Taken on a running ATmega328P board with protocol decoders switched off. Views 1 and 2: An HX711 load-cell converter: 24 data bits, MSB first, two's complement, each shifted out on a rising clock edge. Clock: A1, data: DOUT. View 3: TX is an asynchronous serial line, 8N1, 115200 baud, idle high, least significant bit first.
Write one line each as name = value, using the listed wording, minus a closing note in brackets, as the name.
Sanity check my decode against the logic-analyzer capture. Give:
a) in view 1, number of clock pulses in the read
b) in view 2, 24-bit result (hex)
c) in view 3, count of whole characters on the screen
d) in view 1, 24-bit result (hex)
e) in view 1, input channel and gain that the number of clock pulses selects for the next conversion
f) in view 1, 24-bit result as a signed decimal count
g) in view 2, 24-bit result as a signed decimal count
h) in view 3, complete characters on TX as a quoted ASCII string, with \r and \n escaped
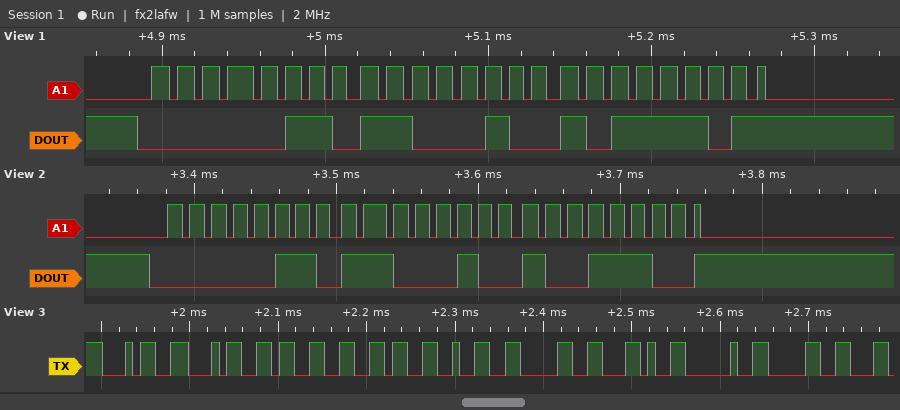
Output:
in view 1, number of clock pulses in the read = 25
in view 2, 24-bit result = 0x06C49C
in view 3, count of whole characters on the screen = 9
in view 1, 24-bit result = 0x06C4BD
in view 1, input channel and gain that the number of clock pulses selects for the next conversion = channel A, gain 128
in view 1, 24-bit result as a signed decimal count = 443581
in view 2, 24-bit result as a signed decimal count = 443548
in view 3, complete characters on TX as a quoted ASCII string, with \r and \n escaped = "443620, 0"
